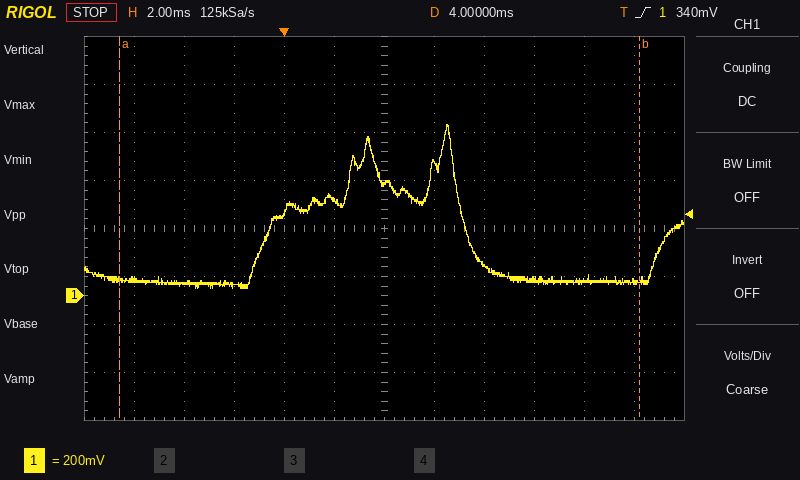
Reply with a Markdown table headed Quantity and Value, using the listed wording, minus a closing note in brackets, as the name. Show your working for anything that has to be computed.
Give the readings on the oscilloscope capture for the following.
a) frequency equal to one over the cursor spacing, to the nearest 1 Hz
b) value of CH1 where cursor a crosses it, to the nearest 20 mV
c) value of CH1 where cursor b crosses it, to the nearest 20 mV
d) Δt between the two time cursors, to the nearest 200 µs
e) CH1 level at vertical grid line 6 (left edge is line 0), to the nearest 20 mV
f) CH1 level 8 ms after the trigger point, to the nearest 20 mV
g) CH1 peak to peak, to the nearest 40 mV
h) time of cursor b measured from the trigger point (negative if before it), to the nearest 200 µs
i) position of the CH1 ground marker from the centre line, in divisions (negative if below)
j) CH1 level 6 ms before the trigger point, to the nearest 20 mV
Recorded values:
| Quantity | Value |
|---|---|
| frequency equal to one over the cursor spacing, to the nearest 1 Hz | 1 / 20.8 ms ≈ 48 Hz |
| value of CH1 where cursor a crosses it, to the nearest 20 mV | 60 mV |
| value of CH1 where cursor b crosses it, to the nearest 20 mV | 60 mV |
| Δt between the two time cursors, to the nearest 200 µs | 20.8 ms |
| CH1 level at vertical grid line 6 (left edge is line 0), to the nearest 20 mV | 460 mV |
| CH1 level 8 ms after the trigger point, to the nearest 20 mV | 120 mV |
| CH1 peak to peak, to the nearest 40 mV | 680 mV |
| time of cursor b measured from the trigger point (negative if before it), to the nearest 200 µs | +14.2 ms |
| position of the CH1 ground marker from the centre line, in divisions | -1.4 div |
| CH1 level 6 ms before the trigger point, to the nearest 20 mV | 60 mV |
